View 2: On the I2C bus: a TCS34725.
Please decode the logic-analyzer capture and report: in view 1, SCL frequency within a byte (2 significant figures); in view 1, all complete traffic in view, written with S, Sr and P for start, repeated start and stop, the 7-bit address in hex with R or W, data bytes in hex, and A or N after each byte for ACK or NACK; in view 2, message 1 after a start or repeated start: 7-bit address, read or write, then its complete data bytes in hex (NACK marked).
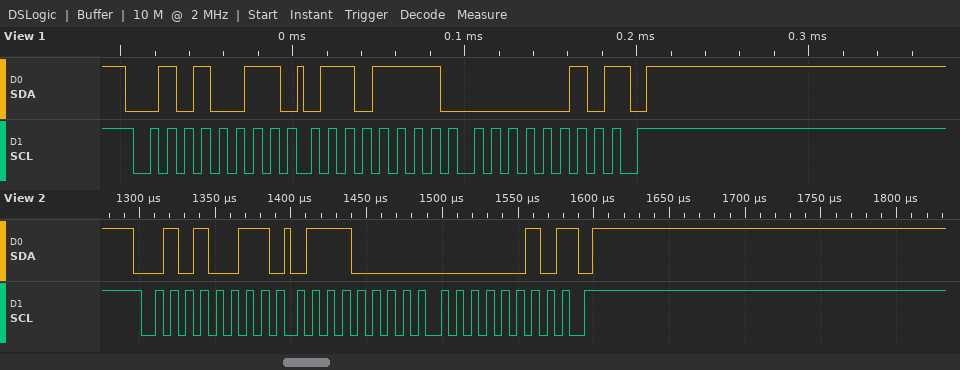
100 kHz
S 29R A 6F A 02 N P
0x29 read: 70 02 NACK
